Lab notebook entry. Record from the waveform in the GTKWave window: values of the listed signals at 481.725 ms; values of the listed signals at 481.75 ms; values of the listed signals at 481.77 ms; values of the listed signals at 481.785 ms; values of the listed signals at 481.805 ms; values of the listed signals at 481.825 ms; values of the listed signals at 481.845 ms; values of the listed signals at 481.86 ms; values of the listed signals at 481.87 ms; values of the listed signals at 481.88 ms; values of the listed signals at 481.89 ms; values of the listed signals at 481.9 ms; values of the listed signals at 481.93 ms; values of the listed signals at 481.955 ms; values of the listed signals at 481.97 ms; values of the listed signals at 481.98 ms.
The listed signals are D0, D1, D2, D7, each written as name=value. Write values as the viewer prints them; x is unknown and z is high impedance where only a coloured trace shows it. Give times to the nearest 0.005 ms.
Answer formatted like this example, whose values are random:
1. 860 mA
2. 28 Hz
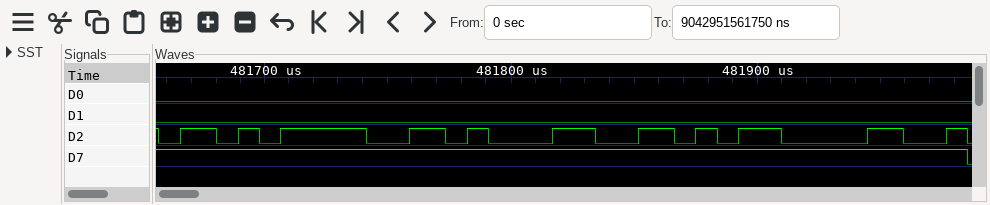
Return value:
1. D0=0, D1=0, D2=1, D7=1
2. D0=0, D1=0, D2=0, D7=1
3. D0=0, D1=0, D2=1, D7=1
4. D0=0, D1=0, D2=1, D7=1
5. D0=0, D1=0, D2=0, D7=1
6. D0=0, D1=0, D2=1, D7=1
7. D0=0, D1=0, D2=0, D7=1
8. D0=0, D1=0, D2=1, D7=1
9. D0=0, D1=0, D2=0, D7=1
10. D0=0, D1=0, D2=1, D7=1
11. D0=0, D1=0, D2=0, D7=1
12. D0=0, D1=0, D2=1, D7=1
13. D0=0, D1=0, D2=0, D7=1
14. D0=0, D1=0, D2=1, D7=1
15. D0=0, D1=0, D2=0, D7=1
16. D0=0, D1=0, D2=1, D7=1
